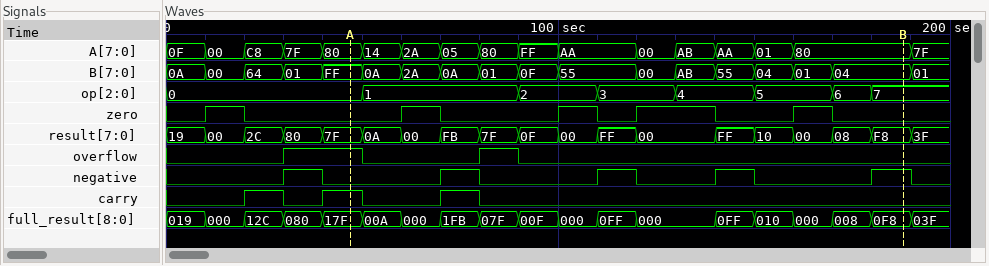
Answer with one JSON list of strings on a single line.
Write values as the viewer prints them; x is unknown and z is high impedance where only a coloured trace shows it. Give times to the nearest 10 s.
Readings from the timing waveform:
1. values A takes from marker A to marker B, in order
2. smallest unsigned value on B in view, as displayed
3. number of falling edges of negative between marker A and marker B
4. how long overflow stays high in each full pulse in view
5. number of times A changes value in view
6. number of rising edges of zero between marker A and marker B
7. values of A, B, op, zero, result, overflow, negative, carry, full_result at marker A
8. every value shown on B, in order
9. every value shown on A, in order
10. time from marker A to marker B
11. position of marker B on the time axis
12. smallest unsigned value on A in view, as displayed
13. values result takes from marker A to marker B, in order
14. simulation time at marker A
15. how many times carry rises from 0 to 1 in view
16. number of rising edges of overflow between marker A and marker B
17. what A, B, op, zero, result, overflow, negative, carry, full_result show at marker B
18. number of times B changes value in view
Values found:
["80, 14, 2A, 05, 80, FF, AA, 00, AB, AA, 01, 80", "00", "3", "20 s, 10 s", "16", "4", "A=80, B=FF, op=0, zero=0, result=7F, overflow=1, negative=0, carry=1, full_result=17F", "0A, 00, 64, 01, FF, 0A, 2A, 0A, 01, 0F, 55, 00, AB, 55, 04, 01, 04, 01", "0F, 00, C8, 7F, 80, 14, 2A, 05, 80, FF, AA, 00, AB, AA, 01, 80, 7F", "140 s", "190 s", "00", "7F, 0A, 00, FB, 7F, 0F, 00, FF, 00, FF, 10, 00, 08, F8", "50 s", "3", "1", "A=80, B=04, op=7, zero=0, result=F8, overflow=0, negative=1, carry=0, full_result=0F8", "17"]
